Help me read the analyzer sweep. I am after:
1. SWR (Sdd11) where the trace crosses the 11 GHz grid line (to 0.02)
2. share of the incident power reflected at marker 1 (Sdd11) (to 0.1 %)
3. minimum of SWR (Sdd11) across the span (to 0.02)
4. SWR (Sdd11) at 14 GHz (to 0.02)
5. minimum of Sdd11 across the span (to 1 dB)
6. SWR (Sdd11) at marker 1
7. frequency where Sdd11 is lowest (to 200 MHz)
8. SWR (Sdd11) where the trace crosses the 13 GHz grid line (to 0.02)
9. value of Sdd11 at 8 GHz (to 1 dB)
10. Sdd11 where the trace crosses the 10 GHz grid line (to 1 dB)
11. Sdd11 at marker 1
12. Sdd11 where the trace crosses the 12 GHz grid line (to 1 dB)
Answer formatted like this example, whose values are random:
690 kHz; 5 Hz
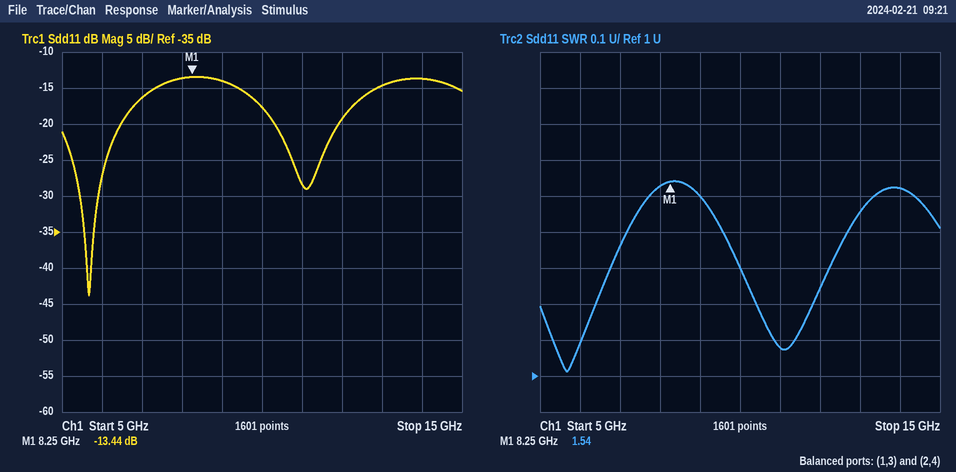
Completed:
1.08; 4.5 %; 1.02; 1.52; -44 dB; 1.54; 5.6 GHz; 1.46; -14 dB; -18 dB; -13.44 dB; -19 dB
